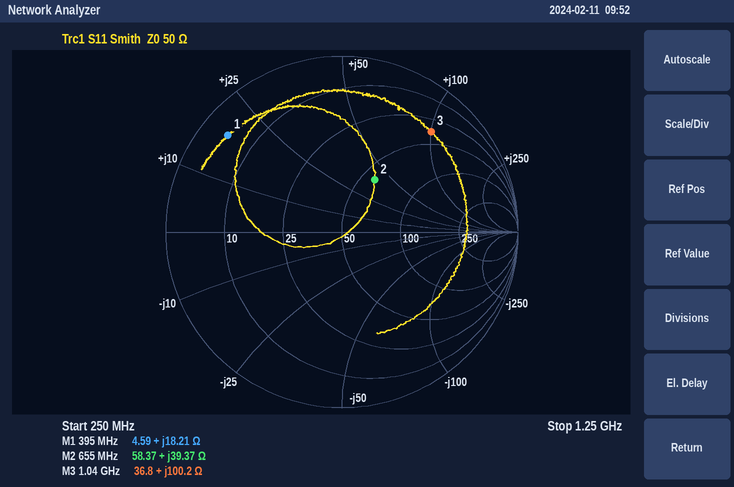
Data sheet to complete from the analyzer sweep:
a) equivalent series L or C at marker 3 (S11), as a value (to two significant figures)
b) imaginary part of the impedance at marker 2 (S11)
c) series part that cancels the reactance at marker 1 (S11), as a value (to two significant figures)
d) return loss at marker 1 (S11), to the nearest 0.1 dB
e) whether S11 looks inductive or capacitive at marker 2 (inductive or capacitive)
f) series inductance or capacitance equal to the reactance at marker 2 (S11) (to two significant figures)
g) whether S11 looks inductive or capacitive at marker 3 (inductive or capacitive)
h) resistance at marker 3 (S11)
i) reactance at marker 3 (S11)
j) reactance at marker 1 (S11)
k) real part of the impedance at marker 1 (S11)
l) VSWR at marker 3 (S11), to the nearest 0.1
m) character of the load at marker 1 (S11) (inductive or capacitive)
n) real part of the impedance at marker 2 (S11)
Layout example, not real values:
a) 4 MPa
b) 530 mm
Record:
a) 15 nH
b) +39.37 Ω
c) 22 pF
d) 1.4 dB
e) inductive
f) 9.6 nH
g) inductive
h) 36.8 Ω
i) +100.2 Ω
j) +18.21 Ω
k) 4.59 Ω
l) 7.4
m) inductive
n) 58.37 Ω
